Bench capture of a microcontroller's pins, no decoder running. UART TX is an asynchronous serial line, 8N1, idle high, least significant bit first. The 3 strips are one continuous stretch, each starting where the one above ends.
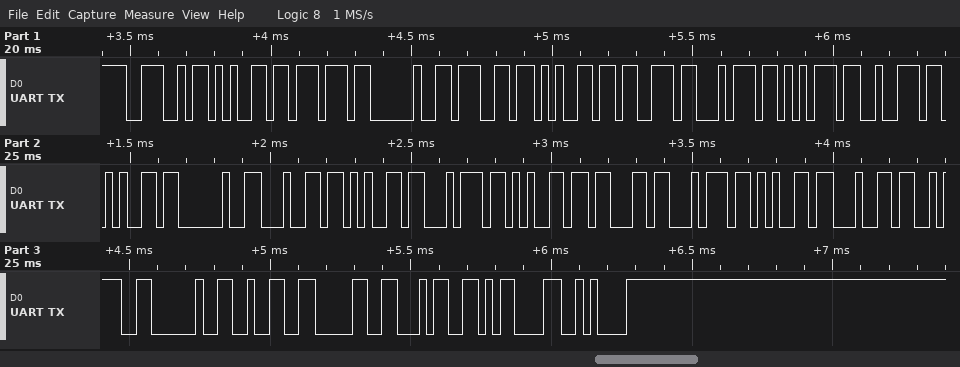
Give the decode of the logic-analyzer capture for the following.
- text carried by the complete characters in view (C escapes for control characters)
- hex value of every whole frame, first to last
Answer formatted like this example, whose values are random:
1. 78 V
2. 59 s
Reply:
1. "New gesture detected: 204\r\n"
2. 4E 65 77 20 67 65 73 74 75 72 65 20 64 65 74 65 63 74 65 64 3A 20 32 30 34 0D 0A
